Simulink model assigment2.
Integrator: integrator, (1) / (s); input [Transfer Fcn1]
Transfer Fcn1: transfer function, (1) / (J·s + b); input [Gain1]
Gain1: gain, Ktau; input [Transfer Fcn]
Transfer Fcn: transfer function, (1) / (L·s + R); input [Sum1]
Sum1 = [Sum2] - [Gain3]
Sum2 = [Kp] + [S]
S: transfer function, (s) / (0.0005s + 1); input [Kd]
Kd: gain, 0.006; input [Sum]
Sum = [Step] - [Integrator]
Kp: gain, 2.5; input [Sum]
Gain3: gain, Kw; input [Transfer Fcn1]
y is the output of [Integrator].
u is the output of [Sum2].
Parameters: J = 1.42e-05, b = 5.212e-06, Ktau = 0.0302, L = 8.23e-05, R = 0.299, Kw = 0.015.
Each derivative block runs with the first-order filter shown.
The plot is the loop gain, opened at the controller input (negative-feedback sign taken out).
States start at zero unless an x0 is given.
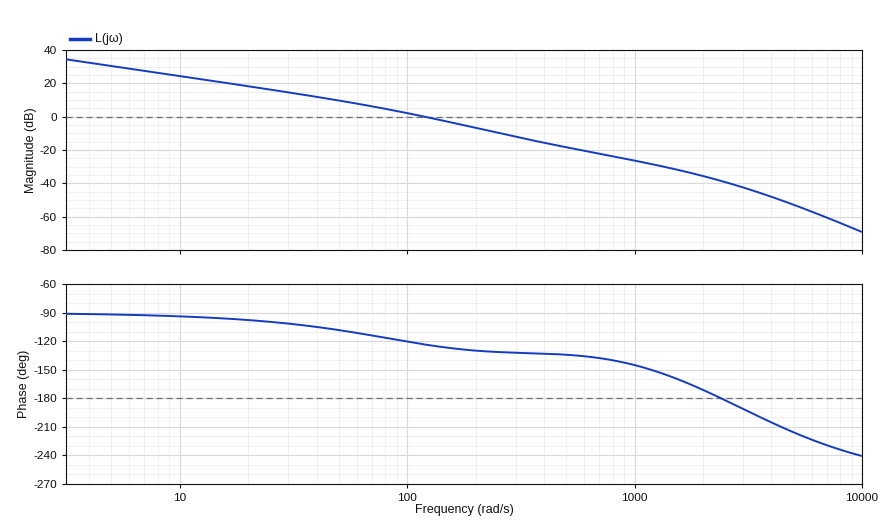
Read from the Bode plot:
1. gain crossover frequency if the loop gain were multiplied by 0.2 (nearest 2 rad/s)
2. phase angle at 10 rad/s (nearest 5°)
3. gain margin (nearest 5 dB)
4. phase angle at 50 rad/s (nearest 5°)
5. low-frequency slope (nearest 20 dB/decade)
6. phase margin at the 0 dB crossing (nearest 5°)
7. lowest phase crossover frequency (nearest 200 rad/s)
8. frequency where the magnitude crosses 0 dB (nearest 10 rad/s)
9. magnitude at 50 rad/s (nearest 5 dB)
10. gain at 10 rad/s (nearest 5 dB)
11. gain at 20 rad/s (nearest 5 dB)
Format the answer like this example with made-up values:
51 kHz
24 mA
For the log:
32 rad/s
-95°
40 dB
-110°
-20 dB/decade
55°
2400 rad/s
120 rad/s
10 dB
25 dB
20 dB
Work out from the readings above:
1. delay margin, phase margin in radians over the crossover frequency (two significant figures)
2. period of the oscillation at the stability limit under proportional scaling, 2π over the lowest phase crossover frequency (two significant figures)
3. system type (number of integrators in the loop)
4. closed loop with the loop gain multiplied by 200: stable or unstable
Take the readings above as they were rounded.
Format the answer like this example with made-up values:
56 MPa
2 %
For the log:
0.0080 s
0.0026 s
1
unstable
